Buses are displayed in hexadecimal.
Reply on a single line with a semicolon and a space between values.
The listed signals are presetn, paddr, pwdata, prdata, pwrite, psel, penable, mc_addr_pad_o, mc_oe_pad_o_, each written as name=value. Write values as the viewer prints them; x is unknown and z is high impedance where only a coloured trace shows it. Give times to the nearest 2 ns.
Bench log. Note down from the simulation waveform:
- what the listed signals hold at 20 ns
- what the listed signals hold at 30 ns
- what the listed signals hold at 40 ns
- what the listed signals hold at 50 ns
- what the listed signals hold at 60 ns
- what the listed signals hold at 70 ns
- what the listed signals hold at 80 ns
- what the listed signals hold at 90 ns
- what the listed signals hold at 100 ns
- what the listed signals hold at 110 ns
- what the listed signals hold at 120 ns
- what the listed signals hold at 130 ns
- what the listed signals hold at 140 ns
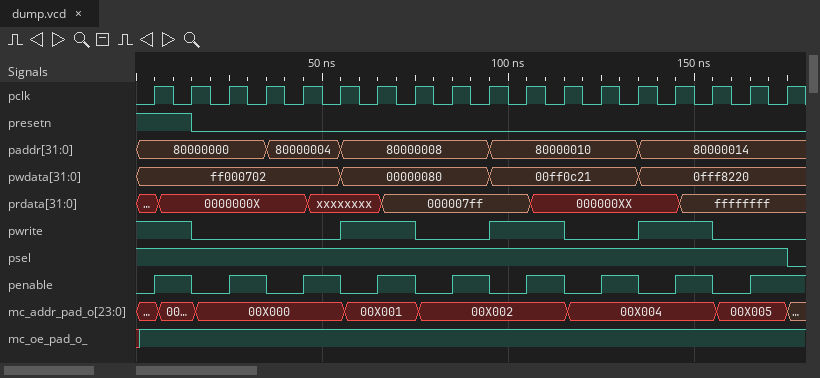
presetn=0, paddr=80000000, pwdata=ff000702, prdata=0000000X, pwrite=0, psel=1, penable=0, mc_addr_pad_o=00X000, mc_oe_pad_o_=1; presetn=0, paddr=80000000, pwdata=ff000702, prdata=0000000X, pwrite=0, psel=1, penable=1, mc_addr_pad_o=00X000, mc_oe_pad_o_=1; presetn=0, paddr=80000004, pwdata=ff000702, prdata=0000000X, pwrite=0, psel=1, penable=0, mc_addr_pad_o=00X000, mc_oe_pad_o_=1; presetn=0, paddr=80000004, pwdata=ff000702, prdata=xxxxxxxx, pwrite=0, psel=1, penable=1, mc_addr_pad_o=00X000, mc_oe_pad_o_=1; presetn=0, paddr=80000008, pwdata=00000080, prdata=xxxxxxxx, pwrite=1, psel=1, penable=0, mc_addr_pad_o=00X001, mc_oe_pad_o_=1; presetn=0, paddr=80000008, pwdata=00000080, prdata=000007ff, pwrite=1, psel=1, penable=1, mc_addr_pad_o=00X001, mc_oe_pad_o_=1; presetn=0, paddr=80000008, pwdata=00000080, prdata=000007ff, pwrite=0, psel=1, penable=0, mc_addr_pad_o=00X002, mc_oe_pad_o_=1; presetn=0, paddr=80000008, pwdata=00000080, prdata=000007ff, pwrite=0, psel=1, penable=1, mc_addr_pad_o=00X002, mc_oe_pad_o_=1; presetn=0, paddr=80000010, pwdata=00ff0c21, prdata=000007ff, pwrite=1, psel=1, penable=0, mc_addr_pad_o=00X002, mc_oe_pad_o_=1; presetn=0, paddr=80000010, pwdata=00ff0c21, prdata=000000XX, pwrite=1, psel=1, penable=1, mc_addr_pad_o=00X002, mc_oe_pad_o_=1; presetn=0, paddr=80000010, pwdata=00ff0c21, prdata=000000XX, pwrite=0, psel=1, penable=0, mc_addr_pad_o=00X004, mc_oe_pad_o_=1; presetn=0, paddr=80000010, pwdata=00ff0c21, prdata=000000XX, pwrite=0, psel=1, penable=1, mc_addr_pad_o=00X004, mc_oe_pad_o_=1; presetn=0, paddr=80000014, pwdata=0fff8220, prdata=000000XX, pwrite=1, psel=1, penable=0, mc_addr_pad_o=00X004, mc_oe_pad_o_=1
